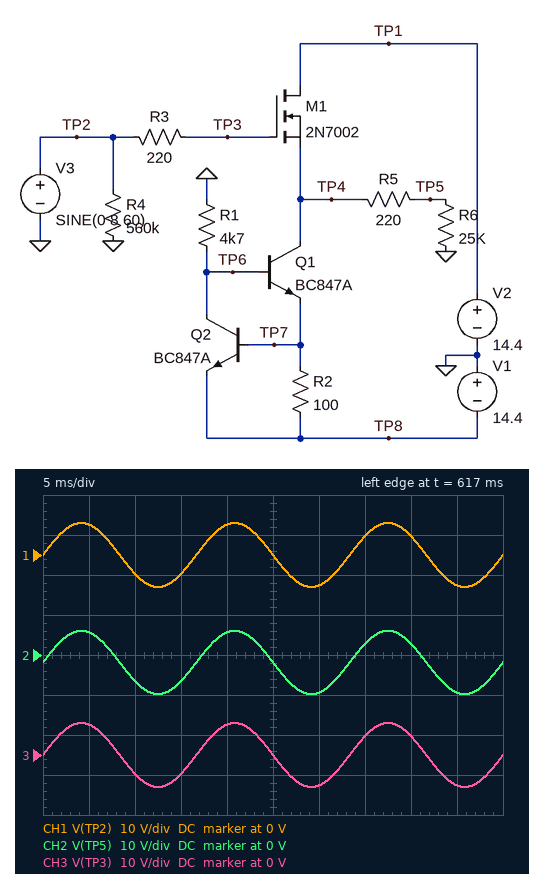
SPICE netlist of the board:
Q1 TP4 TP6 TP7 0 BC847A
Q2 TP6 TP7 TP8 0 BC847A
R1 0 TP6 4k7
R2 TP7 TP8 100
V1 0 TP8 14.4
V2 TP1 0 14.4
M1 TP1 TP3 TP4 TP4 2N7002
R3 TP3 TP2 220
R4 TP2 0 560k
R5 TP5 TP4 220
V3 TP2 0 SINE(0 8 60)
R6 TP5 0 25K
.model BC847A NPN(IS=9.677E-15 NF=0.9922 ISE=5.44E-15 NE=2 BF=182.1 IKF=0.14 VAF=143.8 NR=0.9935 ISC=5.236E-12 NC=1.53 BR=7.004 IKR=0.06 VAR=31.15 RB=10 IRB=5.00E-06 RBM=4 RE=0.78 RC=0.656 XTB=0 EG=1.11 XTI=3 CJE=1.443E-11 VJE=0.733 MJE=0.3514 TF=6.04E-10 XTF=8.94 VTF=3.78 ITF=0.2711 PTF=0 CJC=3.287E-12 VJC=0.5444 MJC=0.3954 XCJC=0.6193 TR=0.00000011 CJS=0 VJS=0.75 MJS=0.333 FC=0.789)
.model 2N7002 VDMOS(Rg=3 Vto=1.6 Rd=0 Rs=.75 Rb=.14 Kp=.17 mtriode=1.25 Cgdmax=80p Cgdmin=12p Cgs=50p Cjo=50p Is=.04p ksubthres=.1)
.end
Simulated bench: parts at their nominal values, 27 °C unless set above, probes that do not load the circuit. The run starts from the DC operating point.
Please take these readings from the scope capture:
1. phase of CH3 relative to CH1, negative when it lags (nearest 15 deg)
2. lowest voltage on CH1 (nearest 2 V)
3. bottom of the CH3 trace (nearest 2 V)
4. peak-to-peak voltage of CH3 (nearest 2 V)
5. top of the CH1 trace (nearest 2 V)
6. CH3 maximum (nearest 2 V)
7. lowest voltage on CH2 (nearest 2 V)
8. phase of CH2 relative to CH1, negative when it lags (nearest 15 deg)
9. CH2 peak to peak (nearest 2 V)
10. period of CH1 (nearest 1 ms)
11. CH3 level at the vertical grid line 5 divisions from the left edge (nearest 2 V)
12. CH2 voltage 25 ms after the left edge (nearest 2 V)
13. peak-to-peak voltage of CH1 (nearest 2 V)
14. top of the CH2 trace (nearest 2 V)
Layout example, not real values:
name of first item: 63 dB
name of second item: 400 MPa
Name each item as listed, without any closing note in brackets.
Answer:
phase of CH3 relative to CH1, negative when it lags: 0 deg
lowest voltage on CH1: -8 V
bottom of the CH3 trace: -8 V
peak-to-peak voltage of CH3: 16 V
top of the CH1 trace: 8 V
CH3 maximum: 8 V
lowest voltage on CH2: -10 V
phase of CH2 relative to CH1, negative when it lags: 0 deg
CH2 peak to peak: 16 V
period of CH1: 17 ms
CH3 level at the vertical grid line 5 divisions from the left edge: 0 V
CH2 voltage 25 ms after the left edge: -2 V
peak-to-peak voltage of CH1: 16 V
top of the CH2 trace: 6 V
